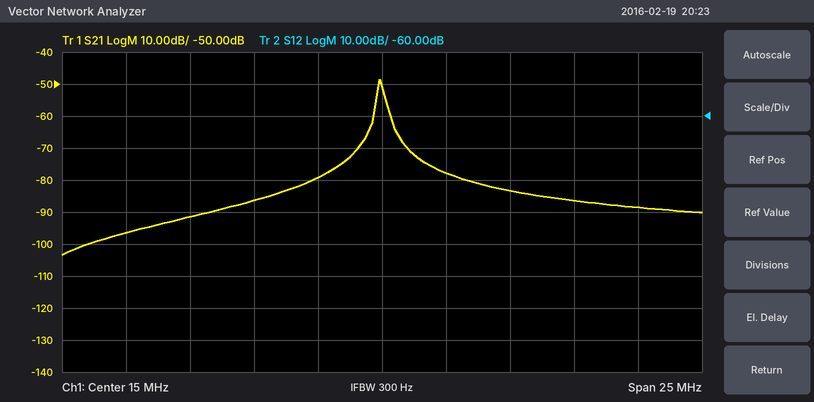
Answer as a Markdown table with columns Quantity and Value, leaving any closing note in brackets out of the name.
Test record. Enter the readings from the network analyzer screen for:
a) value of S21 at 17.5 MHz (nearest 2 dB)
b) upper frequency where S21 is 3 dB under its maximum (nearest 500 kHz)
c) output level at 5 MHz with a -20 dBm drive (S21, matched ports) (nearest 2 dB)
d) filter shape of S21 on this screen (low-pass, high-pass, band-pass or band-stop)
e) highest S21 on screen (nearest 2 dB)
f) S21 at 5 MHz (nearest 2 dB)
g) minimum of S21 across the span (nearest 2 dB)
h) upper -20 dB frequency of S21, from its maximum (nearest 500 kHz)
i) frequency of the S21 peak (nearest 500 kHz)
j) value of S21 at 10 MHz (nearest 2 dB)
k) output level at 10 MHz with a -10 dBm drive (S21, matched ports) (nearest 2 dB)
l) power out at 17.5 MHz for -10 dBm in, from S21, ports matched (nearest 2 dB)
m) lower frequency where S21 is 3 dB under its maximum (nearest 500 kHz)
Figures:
| Quantity | Value |
|---|---|
| value of S21 at 17.5 MHz | -78 dB |
| upper frequency where S21 is 3 dB under its maximum | 15.0 MHz |
| output level at 5 MHz with a -20 dBm drive (S21, matched ports) | -116 dBm |
| filter shape of S21 on this screen | band-pass |
| highest S21 on screen | -48 dB |
| S21 at 5 MHz | -96 dB |
| minimum of S21 across the span | -104 dB |
| upper -20 dB frequency of S21, from its maximum | 16.0 MHz |
| frequency of the S21 peak | 15.0 MHz |
| value of S21 at 10 MHz | -86 dB |
| output level at 10 MHz with a -10 dBm drive (S21, matched ports) | -96 dBm |
| power out at 17.5 MHz for -10 dBm in, from S21, ports matched | -88 dBm |
| lower frequency where S21 is 3 dB under its maximum | 15.0 MHz |
